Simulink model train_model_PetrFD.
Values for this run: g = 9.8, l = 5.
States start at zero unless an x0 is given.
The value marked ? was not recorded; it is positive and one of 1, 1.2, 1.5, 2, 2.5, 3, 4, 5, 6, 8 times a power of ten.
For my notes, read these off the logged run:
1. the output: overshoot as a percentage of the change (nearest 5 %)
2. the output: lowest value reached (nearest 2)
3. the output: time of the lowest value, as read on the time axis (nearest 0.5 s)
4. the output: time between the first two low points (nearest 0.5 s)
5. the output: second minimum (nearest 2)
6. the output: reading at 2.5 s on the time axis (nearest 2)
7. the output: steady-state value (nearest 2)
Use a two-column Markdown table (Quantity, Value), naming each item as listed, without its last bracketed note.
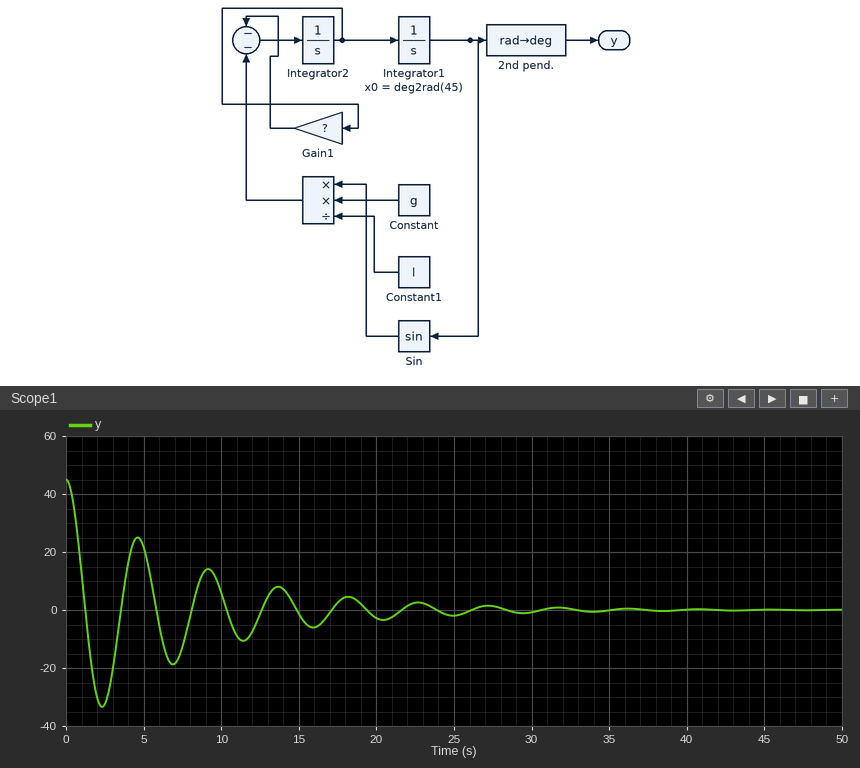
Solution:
| Quantity | Value |
|---|---|
| the output: overshoot as a percentage of the change | 75 % |
| the output: lowest value reached | -34 |
| the output: time of the lowest value, as read on the time axis | 2.5 s |
| the output: time between the first two low points | 4.5 s |
| the output: second minimum | -18 |
| the output: reading at 2.5 s on the time axis | -32 |
| the output: steady-state value | 0 |
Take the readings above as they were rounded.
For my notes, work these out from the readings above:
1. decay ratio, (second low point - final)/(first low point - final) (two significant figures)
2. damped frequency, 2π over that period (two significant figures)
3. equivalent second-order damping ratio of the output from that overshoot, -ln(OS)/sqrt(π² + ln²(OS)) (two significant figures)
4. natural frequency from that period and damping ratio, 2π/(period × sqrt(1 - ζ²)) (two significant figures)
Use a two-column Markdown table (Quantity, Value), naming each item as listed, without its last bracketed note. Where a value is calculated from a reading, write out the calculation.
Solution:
| Quantity | Value |
|---|---|
| decay ratio, (second low point - final)/(first low point - final) | (-18 - 0) / (-34 - 0) = 0.53 |
| damped frequency, 2π over that period | 2π / 4.5 = 1.4 rad/s |
| equivalent second-order damping ratio of the output from that overshoot, -ln(OS)/sqrt(π² + ln²(OS)) | ln(0.75) = -0.288; 0.288 / sqrt(9.870 + 0.083) = 0.091 |
| natural frequency from that period and damping ratio, 2π/(period × sqrt(1 - ζ²)) | 2π / (4.5 × sqrt(1 - 0.091²)) = 1.4 rad/s |
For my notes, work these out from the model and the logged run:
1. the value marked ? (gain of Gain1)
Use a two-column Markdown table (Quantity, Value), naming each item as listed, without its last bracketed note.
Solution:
| Quantity | Value |
|---|---|
| the value marked ? | 0.25 |
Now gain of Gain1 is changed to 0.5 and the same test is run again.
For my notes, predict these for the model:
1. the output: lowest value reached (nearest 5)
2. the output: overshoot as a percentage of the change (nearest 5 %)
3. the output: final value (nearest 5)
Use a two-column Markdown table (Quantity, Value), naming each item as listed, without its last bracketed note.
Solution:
| Quantity | Value |
|---|---|
| the output: lowest value reached | -25 |
| the output: overshoot as a percentage of the change | 55 % |
| the output: final value | 0 |
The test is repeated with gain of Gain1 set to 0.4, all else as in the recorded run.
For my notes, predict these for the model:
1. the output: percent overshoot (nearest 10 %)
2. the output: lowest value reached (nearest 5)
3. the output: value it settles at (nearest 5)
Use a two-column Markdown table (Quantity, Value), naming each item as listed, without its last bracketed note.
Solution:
| Quantity | Value |
|---|---|
| the output: percent overshoot | 60 % |
| the output: lowest value reached | -30 |
| the output: value it settles at | 0 |
